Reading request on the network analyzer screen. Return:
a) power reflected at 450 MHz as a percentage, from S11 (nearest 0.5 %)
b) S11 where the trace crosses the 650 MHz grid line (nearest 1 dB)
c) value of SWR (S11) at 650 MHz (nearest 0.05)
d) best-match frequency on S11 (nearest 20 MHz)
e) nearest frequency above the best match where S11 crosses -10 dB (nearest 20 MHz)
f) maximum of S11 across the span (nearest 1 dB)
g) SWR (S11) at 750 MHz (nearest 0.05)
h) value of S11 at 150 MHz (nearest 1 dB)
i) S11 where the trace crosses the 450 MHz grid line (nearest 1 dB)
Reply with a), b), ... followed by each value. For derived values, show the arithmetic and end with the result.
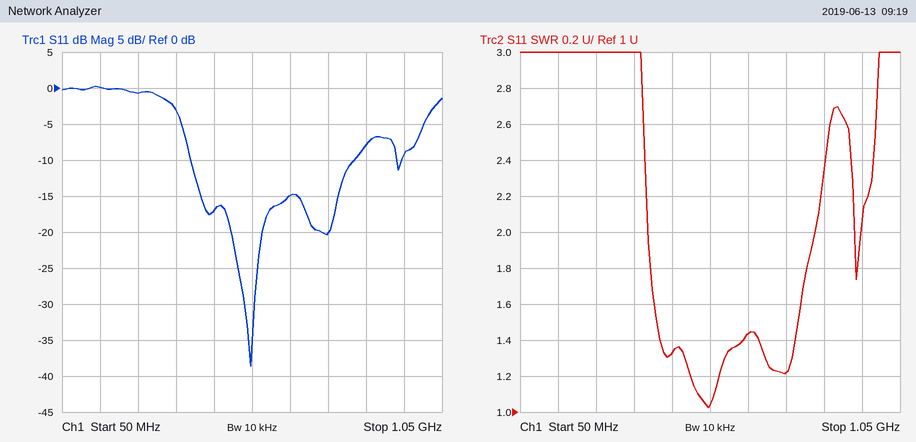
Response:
a) 10^(-17/10) ≈ 2.0 %
b) -15 dB
c) 1.45
d) 540 MHz
e) 820 MHz
f) 0 dB
g) 1.20
h) 0 dB
i) -17 dB
